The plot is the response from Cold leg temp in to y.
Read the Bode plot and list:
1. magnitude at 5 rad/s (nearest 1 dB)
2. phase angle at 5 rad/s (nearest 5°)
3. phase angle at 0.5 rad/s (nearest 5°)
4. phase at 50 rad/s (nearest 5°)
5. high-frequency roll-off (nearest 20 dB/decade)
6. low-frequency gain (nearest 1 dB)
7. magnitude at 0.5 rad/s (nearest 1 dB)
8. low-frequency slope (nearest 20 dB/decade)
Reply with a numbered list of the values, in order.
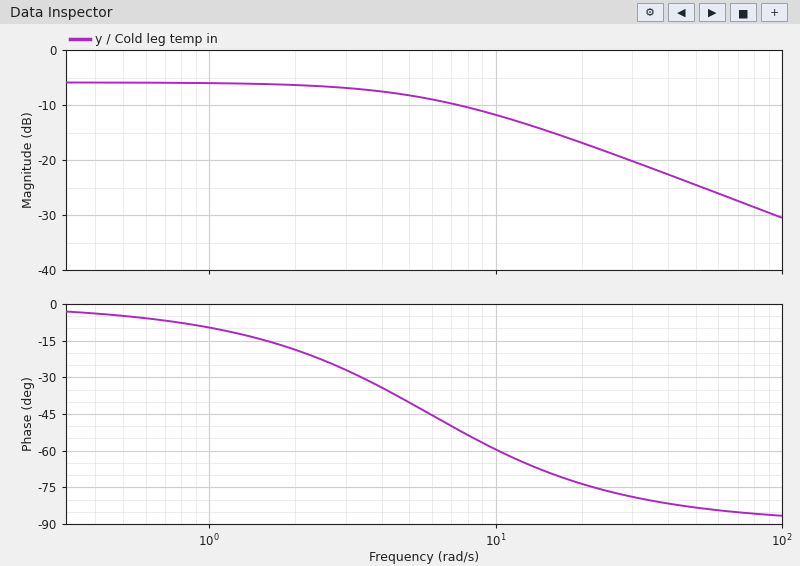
1. -8 dB
2. -40°
3. -5°
4. -85°
5. -20 dB/decade
6. -6 dB
7. -6 dB
8. 0 dB/decade
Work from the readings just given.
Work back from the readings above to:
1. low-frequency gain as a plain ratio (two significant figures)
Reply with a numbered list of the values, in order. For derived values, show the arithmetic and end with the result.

1. 10^(-6 / 20) = 0.50
